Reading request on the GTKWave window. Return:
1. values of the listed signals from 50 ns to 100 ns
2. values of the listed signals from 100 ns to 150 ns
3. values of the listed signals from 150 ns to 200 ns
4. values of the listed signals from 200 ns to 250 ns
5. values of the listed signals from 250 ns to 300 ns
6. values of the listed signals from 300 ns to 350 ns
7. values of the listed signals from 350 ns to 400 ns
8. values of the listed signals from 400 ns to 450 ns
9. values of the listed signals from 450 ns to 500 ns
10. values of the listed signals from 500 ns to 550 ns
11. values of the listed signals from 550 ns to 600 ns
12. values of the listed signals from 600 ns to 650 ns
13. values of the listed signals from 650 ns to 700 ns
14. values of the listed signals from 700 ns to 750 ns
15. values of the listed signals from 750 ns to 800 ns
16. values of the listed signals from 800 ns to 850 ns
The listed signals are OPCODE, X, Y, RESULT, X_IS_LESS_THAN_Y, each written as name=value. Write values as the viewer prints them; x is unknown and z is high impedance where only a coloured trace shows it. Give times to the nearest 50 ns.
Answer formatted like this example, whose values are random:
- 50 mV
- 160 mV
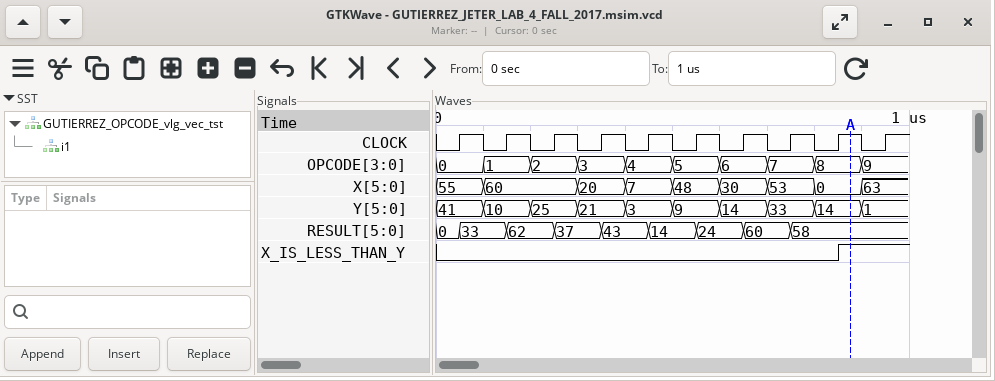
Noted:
- OPCODE=0, X=55, Y=41, RESULT=33, X_IS_LESS_THAN_Y=0
- OPCODE=1, X=60, Y=10, RESULT=33, X_IS_LESS_THAN_Y=0
- OPCODE=1, X=60, Y=10, RESULT=62, X_IS_LESS_THAN_Y=0
- OPCODE=2, X=60, Y=25, RESULT=62, X_IS_LESS_THAN_Y=0
- OPCODE=2, X=60, Y=25, RESULT=37, X_IS_LESS_THAN_Y=0
- OPCODE=3, X=20, Y=21, RESULT=37, X_IS_LESS_THAN_Y=0
- OPCODE=3, X=20, Y=21, RESULT=43, X_IS_LESS_THAN_Y=0
- OPCODE=4, X=7, Y=3, RESULT=43, X_IS_LESS_THAN_Y=0
- OPCODE=4, X=7, Y=3, RESULT=14, X_IS_LESS_THAN_Y=0
- OPCODE=5, X=48, Y=9, RESULT=14, X_IS_LESS_THAN_Y=0
- OPCODE=5, X=48, Y=9, RESULT=24, X_IS_LESS_THAN_Y=0
- OPCODE=6, X=30, Y=14, RESULT=24, X_IS_LESS_THAN_Y=0
- OPCODE=6, X=30, Y=14, RESULT=60, X_IS_LESS_THAN_Y=0
- OPCODE=7, X=53, Y=33, RESULT=60, X_IS_LESS_THAN_Y=0
- OPCODE=7, X=53, Y=33, RESULT=58, X_IS_LESS_THAN_Y=0
- OPCODE=8, X=0, Y=14, RESULT=58, X_IS_LESS_THAN_Y=0
